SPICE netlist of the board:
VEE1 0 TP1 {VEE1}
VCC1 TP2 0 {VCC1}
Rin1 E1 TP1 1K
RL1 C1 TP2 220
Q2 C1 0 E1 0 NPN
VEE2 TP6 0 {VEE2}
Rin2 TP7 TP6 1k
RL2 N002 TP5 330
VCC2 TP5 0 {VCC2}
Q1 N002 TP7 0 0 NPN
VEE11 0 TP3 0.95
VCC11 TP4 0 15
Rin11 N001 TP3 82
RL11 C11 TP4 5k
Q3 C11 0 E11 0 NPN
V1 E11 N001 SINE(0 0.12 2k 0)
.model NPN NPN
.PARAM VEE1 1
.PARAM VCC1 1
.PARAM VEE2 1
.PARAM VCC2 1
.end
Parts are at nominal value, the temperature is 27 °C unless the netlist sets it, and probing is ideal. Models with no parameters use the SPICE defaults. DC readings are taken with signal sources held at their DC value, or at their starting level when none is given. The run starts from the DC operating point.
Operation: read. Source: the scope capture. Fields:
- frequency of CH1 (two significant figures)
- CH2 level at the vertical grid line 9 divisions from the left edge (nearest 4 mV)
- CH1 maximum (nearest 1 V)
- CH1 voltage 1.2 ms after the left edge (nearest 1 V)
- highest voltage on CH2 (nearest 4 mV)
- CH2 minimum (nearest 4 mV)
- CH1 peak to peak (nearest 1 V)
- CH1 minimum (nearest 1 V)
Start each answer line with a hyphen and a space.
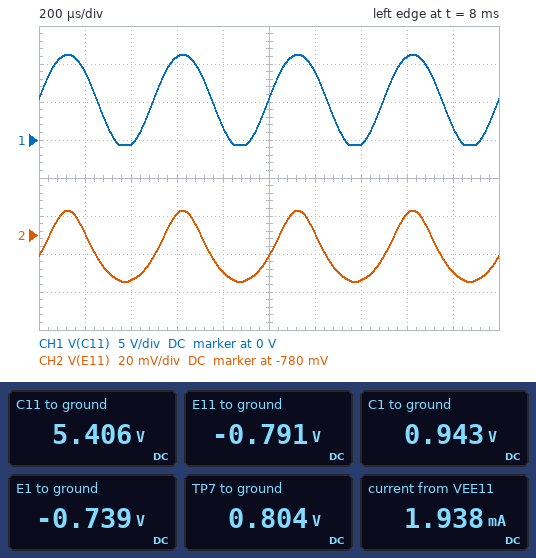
- 2.0 kHz
- -800 mV
- 11 V
- 9 V
- -768 mV
- -804 mV
- 12 V
- -1 V
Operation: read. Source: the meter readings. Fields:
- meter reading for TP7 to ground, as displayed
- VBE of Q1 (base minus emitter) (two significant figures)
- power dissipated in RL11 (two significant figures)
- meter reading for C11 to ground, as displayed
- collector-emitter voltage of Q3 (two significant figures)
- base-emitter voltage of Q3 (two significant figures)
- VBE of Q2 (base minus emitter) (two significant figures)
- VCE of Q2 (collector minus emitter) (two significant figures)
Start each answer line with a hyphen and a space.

- 0.804 V
- 800 mV
- 18 mW
- 5.406 V
- 6.2 V
- 790 mV
- 740 mV
- 1.7 V
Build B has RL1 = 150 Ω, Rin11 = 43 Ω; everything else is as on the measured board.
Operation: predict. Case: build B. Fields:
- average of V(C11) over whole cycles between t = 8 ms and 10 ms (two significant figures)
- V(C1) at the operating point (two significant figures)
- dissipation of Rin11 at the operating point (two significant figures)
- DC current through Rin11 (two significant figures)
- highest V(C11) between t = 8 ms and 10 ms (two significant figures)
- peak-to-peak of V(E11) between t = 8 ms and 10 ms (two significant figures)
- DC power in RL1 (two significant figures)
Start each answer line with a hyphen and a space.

- 2.3 V
- 960 mV
- 480 µW
- 3.3 mA
- 9.1 V
- 49 mV
- 10 µW
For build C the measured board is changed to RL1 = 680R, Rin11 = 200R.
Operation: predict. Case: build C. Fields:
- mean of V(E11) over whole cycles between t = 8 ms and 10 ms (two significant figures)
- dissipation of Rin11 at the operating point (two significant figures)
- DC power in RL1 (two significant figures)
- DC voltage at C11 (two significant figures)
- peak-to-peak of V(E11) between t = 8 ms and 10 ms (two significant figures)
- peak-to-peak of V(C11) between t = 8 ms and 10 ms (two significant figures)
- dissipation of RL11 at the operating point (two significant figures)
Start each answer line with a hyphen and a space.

- -770 mV
- 160 µW
- 45 µW
- 11 V
- 33 mV
- 5.1 V
- 3.9 mW
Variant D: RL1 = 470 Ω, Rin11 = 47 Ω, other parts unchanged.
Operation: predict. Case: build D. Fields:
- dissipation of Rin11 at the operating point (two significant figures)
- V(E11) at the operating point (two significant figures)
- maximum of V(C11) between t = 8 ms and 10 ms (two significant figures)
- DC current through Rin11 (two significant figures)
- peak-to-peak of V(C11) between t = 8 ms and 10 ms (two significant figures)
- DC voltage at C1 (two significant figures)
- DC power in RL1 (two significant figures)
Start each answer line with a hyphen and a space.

- 460 µW
- -800 mV
- 9.4 V
- 3.1 mA
- 10 V
- 880 mV
- 31 µW
